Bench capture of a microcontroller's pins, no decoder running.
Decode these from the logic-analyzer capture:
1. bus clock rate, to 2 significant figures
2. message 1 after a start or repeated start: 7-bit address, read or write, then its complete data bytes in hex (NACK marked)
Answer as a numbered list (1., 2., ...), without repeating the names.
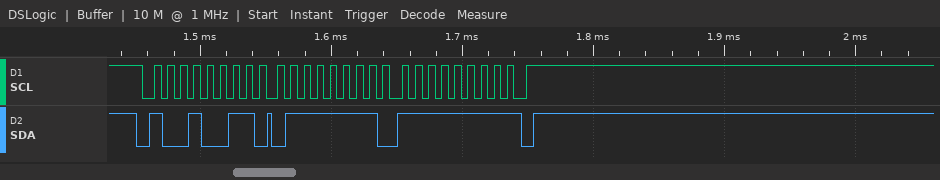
1. 100 kHz
2. 0x49 read: 7F FF NACK
